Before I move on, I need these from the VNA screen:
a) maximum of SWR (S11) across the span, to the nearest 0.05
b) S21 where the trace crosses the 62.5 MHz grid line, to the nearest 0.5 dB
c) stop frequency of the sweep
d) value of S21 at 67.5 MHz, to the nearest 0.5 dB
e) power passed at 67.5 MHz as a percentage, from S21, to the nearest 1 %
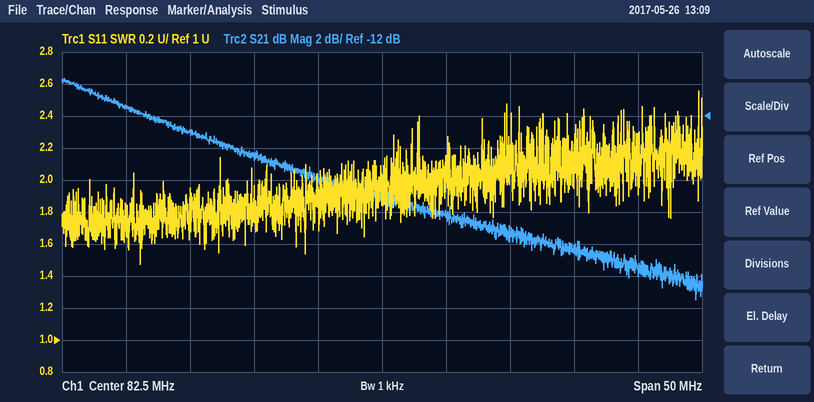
2.55
-11.5 dB
107.5 MHz
-13.0 dB
5 %
